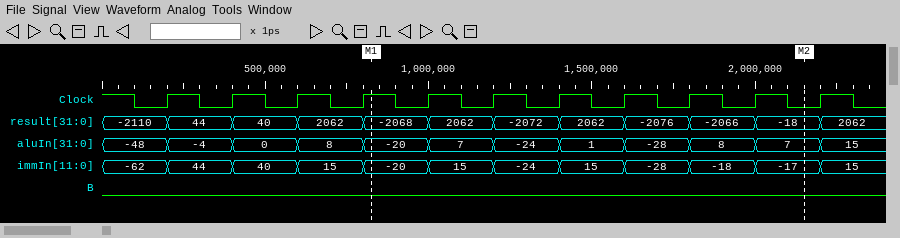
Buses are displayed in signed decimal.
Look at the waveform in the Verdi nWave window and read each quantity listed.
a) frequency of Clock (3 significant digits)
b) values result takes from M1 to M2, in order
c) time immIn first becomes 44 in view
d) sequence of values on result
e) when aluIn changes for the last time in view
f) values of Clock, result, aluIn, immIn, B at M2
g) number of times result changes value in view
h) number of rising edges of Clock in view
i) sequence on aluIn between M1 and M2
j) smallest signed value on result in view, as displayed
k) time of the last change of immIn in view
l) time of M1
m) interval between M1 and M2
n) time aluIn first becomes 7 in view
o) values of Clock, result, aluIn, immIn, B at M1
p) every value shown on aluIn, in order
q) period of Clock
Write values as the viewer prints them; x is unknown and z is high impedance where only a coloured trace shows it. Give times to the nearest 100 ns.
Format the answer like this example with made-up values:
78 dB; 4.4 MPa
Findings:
5.00 MHz; -2068, 2062, -2072, 2062, -2076, -2066, -18; 200 ns; -2110, 44, 40, 2062, -2068, 2062, -2072, 2062, -2076, -2066, -18, 2062; 2200 ns; Clock=0, result=-18, aluIn=7, immIn=-17, B=0; 11; 11; -20, 7, -24, 1, -28, 8, 7; -2110; 2200 ns; 800 ns; 1300 ns; 1000 ns; Clock=1, result=-2068, aluIn=-20, immIn=-20, B=0; -48, -4, 0, 8, -20, 7, -24, 1, -28, 8, 7, 15; 200 ns
